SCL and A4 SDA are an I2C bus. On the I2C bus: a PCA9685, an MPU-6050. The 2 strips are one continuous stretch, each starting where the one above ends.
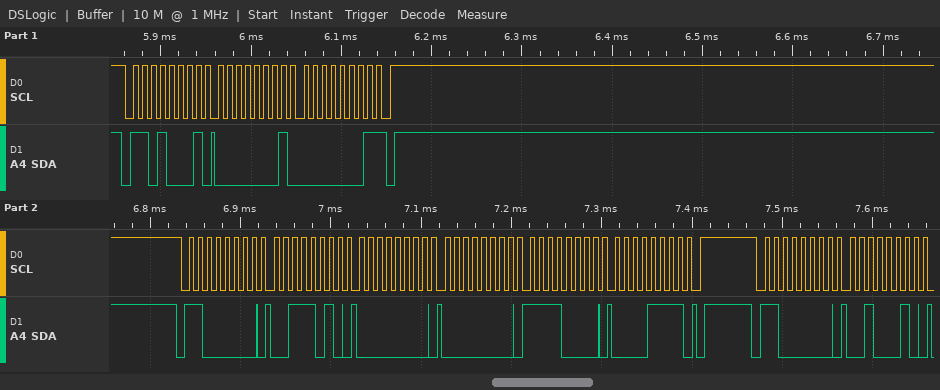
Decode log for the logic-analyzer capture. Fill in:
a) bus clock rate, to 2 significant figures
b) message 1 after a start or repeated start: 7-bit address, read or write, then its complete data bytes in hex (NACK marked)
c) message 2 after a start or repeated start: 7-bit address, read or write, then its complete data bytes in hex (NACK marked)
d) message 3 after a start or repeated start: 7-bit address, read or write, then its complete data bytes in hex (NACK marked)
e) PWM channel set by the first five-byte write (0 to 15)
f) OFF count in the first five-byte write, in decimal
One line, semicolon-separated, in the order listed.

100 kHz; 0x68 read: 01 01 NACK; 0x60 write: 3A 00 00 F0 0F; 0x60 write: 22; 13; 4080
